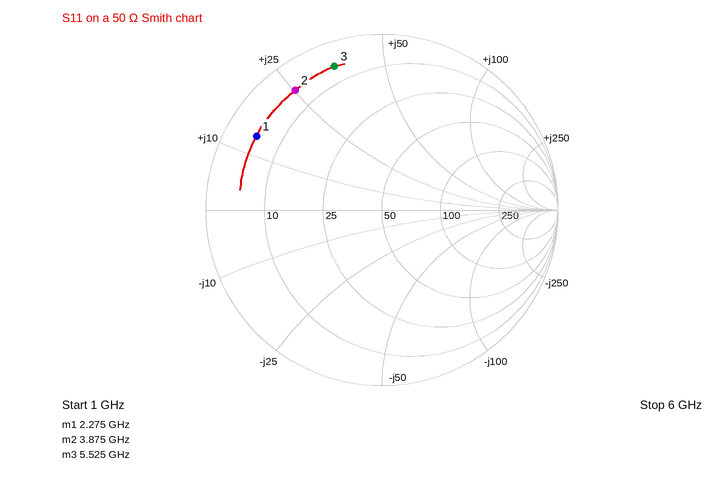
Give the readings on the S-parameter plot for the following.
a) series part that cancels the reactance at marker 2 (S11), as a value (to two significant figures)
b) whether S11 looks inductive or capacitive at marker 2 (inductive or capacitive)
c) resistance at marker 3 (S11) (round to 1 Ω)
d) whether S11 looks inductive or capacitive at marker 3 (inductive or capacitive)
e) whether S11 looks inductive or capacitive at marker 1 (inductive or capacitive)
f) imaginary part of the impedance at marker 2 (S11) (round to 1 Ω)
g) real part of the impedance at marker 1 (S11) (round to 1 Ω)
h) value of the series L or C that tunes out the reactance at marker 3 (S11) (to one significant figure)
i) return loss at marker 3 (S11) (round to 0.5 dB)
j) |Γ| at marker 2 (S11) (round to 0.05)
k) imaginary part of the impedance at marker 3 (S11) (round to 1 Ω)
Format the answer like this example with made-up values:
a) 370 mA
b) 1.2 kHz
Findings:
a) 1.6 pF
b) inductive
c) 6 Ω
d) inductive
e) inductive
f) +25 Ω
g) 5 Ω
h) 800 fF
i) 1.5 dB
j) 0.85
k) +36 Ω
